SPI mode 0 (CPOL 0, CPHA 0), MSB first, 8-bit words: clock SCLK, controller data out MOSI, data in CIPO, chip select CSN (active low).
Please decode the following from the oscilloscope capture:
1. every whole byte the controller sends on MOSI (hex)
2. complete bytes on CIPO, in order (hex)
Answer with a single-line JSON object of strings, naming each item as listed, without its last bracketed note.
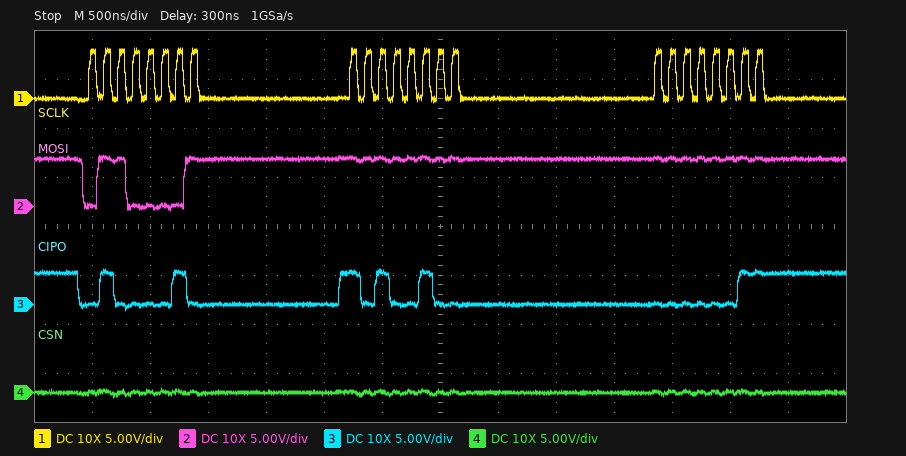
{"every whole byte the controller sends on MOSI": "0x61 0xFF 0xFF", "complete bytes on CIPO, in order": "0x42 0xA4 0x03"}
